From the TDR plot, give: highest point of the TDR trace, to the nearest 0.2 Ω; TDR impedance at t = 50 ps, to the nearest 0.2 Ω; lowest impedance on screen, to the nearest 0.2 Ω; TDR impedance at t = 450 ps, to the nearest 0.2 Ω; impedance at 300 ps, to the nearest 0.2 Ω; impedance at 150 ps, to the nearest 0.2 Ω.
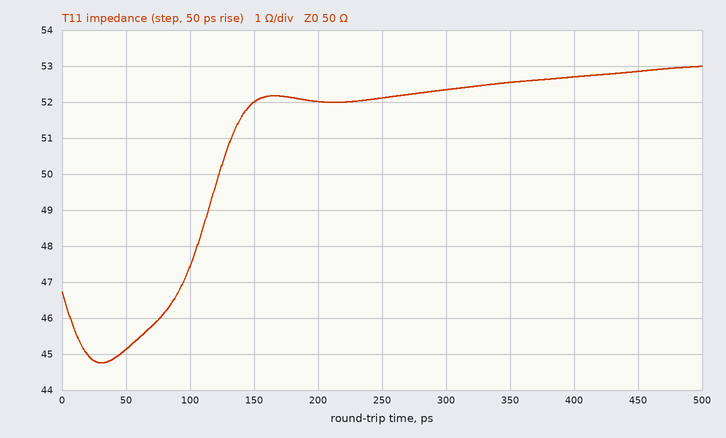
53.0 Ω
45.2 Ω
44.8 Ω
52.8 Ω
52.4 Ω
52.0 Ω
